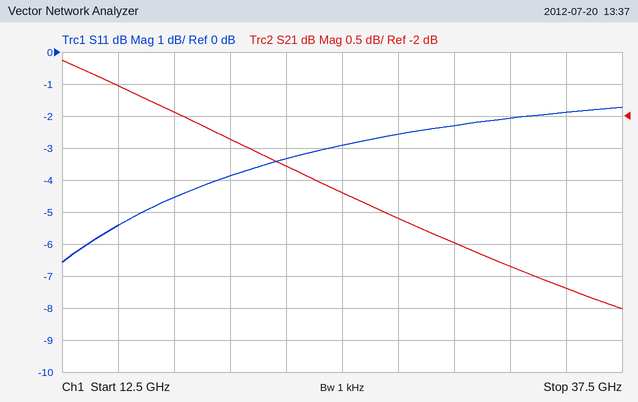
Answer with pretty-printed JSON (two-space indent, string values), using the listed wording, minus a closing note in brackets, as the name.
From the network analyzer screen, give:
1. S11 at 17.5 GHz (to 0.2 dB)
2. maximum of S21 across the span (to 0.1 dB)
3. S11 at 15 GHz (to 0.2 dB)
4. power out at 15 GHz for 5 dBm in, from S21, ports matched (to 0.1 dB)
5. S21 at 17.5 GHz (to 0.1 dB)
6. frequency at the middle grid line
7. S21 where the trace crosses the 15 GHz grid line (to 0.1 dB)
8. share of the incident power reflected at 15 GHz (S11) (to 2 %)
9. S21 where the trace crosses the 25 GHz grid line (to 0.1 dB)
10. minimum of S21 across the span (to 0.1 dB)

{
  "S11 at 17.5 GHz": "-4.6 dB",
  "maximum of S21 across the span": "-1.1 dB",
  "S11 at 15 GHz": "-5.4 dB",
  "power out at 15 GHz for 5 dBm in, from S21, ports matched": "3.5 dBm",
  "S21 at 17.5 GHz": "-1.9 dB",
  "frequency at the middle grid line": "25 GHz",
  "S21 where the trace crosses the 15 GHz grid line": "-1.5 dB",
  "share of the incident power reflected at 15 GHz (S11)": "28 %",
  "S21 where the trace crosses the 25 GHz grid line": "-3.2 dB",
  "minimum of S21 across the span": "-5.0 dB"
}
